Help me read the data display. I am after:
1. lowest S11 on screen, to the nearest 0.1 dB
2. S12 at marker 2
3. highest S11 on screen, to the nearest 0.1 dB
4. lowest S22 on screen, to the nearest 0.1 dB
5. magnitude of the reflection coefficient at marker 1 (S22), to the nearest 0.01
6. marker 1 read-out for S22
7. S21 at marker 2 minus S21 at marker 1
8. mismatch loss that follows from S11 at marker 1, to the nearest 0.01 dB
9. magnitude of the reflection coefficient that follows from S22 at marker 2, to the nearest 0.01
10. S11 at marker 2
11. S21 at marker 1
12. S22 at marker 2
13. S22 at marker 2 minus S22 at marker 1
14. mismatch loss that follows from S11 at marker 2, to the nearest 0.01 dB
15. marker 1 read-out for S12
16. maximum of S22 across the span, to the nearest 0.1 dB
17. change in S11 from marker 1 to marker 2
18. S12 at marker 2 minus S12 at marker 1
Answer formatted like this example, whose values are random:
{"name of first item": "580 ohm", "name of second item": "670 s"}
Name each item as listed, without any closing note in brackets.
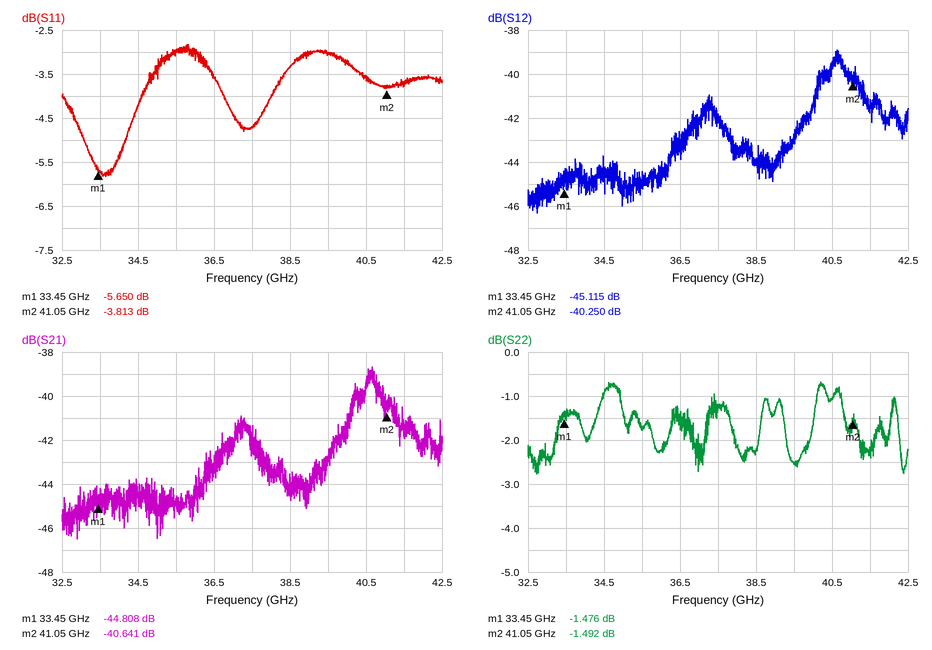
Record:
{"lowest S11 on screen, to the nearest 0.1 dB": "-5.8 dB", "S12 at marker 2": "-40.250 dB", "highest S11 on screen, to the nearest 0.1 dB": "-2.8 dB", "lowest S22 on screen, to the nearest 0.1 dB": "-2.8 dB", "magnitude of the reflection coefficient at marker 1 (S22), to the nearest 0.01": "0.84", "marker 1 read-out for S22": "-1.476 dB", "S21 at marker 2 minus S21 at marker 1": "4.167 dB", "mismatch loss that follows from S11 at marker 1, to the nearest 0.01 dB": "1.38 dB", "magnitude of the reflection coefficient that follows from S22 at marker 2, to the nearest 0.01": "0.84", "S11 at marker 2": "-3.813 dB", "S21 at marker 1": "-44.808 dB", "S22 at marker 2": "-1.492 dB", "S22 at marker 2 minus S22 at marker 1": "-0.016 dB", "mismatch loss that follows from S11 at marker 2, to the nearest 0.01 dB": "2.33 dB", "marker 1 read-out for S12": "-45.115 dB", "maximum of S22 across the span, to the nearest 0.1 dB": "-0.7 dB", "change in S11 from marker 1 to marker 2": "1.837 dB", "S12 at marker 2 minus S12 at marker 1": "4.865 dB"}
